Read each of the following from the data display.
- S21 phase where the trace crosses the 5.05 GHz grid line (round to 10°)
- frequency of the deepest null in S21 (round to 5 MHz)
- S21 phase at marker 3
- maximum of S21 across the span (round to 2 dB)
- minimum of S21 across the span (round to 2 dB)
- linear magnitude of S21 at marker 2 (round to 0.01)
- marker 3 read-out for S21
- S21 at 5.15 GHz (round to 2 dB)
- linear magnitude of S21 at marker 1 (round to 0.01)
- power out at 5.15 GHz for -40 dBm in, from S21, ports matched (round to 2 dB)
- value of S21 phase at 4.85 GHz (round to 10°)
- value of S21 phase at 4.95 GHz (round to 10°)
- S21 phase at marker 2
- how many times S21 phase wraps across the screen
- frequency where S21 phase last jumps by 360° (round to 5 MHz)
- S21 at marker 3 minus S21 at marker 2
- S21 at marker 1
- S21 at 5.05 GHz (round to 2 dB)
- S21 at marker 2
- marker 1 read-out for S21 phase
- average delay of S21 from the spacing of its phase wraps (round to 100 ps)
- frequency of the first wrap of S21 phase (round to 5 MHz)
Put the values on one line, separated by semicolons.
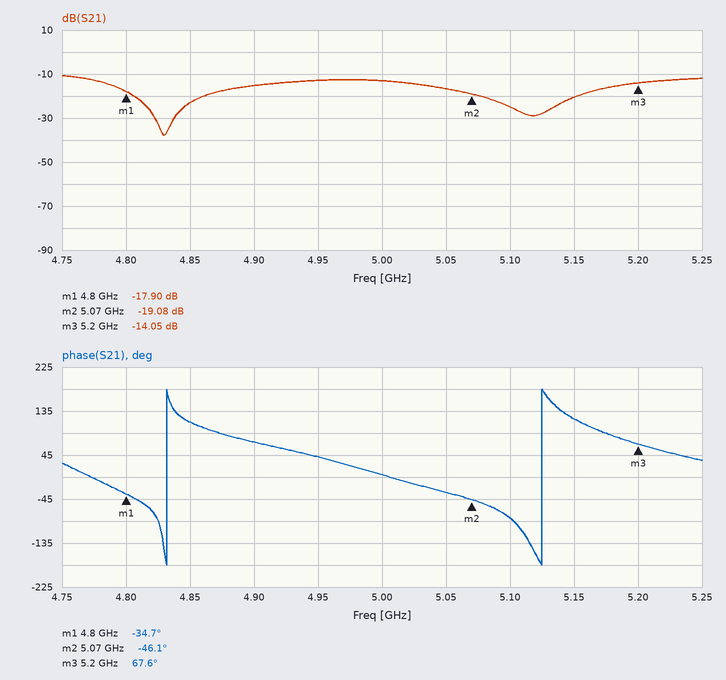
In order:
-30°; 4.830 GHz; 67.6°; -10 dB; -38 dB; 0.11; -14.05 dB; -20 dB; 0.13; -60 dBm; 110°; 40°; -46.1°; 2; 5.125 GHz; 5.03 dB; -17.90 dB; -16 dB; -19.08 dB; -34.7°; 3.4 ns; 4.830 GHz
